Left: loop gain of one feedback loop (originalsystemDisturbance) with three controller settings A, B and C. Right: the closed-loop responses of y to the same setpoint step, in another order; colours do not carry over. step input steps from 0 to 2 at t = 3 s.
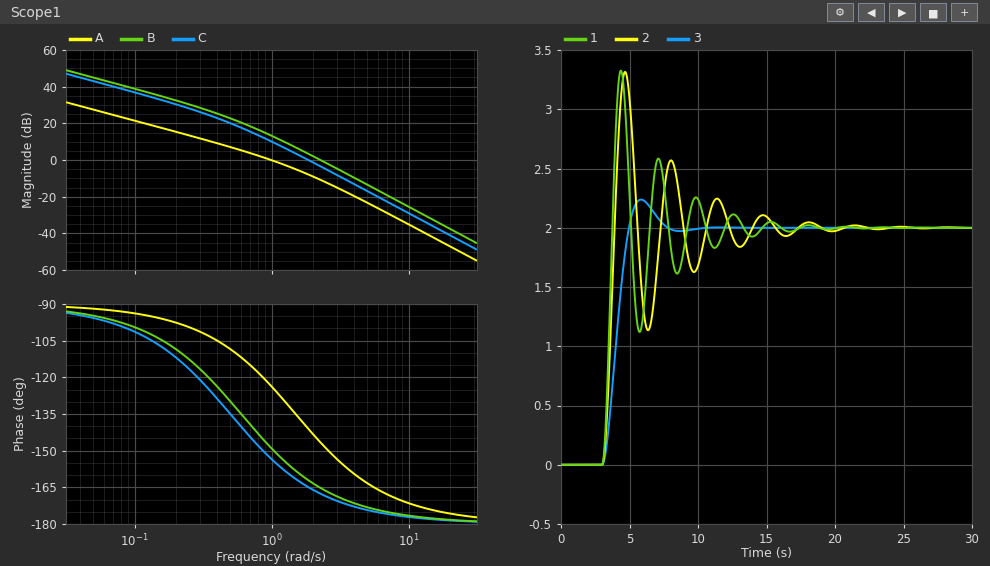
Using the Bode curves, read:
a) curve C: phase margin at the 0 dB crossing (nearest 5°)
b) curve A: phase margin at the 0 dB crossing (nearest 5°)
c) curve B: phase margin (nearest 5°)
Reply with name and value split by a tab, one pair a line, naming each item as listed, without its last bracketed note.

curve C: phase margin at the 0 dB crossing	15°
curve A: phase margin at the 0 dB crossing	55°
curve B: phase margin	15°
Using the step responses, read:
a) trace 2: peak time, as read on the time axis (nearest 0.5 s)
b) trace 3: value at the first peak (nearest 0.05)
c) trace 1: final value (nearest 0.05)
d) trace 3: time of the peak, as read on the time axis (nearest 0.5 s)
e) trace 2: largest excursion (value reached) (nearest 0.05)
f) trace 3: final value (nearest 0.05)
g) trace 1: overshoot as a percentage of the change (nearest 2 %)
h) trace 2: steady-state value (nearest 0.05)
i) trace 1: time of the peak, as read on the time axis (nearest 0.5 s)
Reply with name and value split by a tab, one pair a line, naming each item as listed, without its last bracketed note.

trace 2: peak time, as read on the time axis	4.5 s
trace 3: value at the first peak	2.25
trace 1: final value	2.00
trace 3: time of the peak, as read on the time axis	6.0 s
trace 2: largest excursion (value reached)	3.30
trace 3: final value	2.00
trace 1: overshoot as a percentage of the change	66 %
trace 2: steady-state value	2.00
trace 1: time of the peak, as read on the time axis	4.5 s
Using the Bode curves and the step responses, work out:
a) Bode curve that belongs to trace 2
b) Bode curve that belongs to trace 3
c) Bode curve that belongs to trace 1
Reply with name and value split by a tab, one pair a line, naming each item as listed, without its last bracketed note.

Bode curve that belongs to trace 2	C
Bode curve that belongs to trace 3	A
Bode curve that belongs to trace 1	B
